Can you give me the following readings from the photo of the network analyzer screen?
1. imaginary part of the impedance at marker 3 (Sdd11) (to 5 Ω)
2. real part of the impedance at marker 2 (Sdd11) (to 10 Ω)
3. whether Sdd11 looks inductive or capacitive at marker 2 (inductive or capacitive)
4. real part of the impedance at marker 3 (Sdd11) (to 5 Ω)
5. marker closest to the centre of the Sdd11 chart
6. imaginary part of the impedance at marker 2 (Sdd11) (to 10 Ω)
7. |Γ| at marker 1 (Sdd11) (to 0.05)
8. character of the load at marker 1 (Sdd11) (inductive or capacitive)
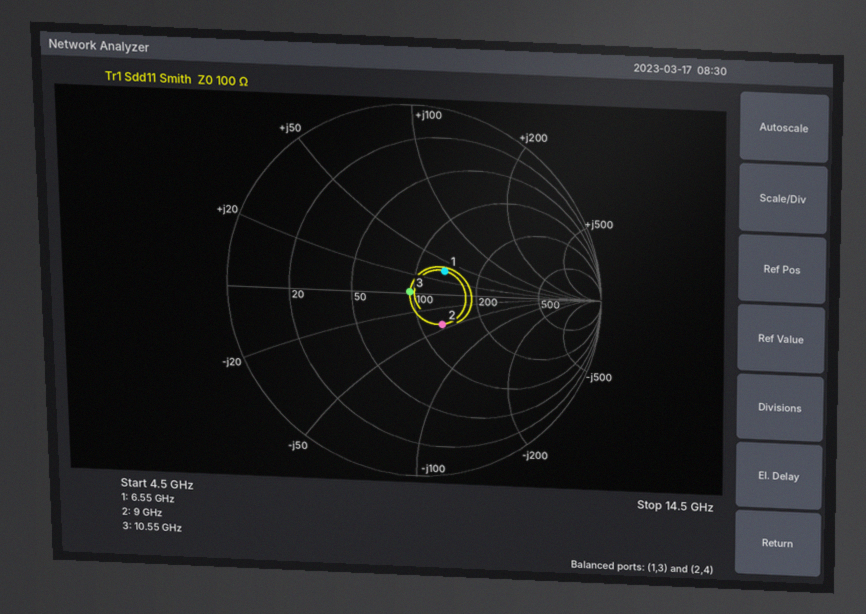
0 Ω
130 Ω
capacitive
95 Ω
marker 3
-40 Ω
0.20
inductive
